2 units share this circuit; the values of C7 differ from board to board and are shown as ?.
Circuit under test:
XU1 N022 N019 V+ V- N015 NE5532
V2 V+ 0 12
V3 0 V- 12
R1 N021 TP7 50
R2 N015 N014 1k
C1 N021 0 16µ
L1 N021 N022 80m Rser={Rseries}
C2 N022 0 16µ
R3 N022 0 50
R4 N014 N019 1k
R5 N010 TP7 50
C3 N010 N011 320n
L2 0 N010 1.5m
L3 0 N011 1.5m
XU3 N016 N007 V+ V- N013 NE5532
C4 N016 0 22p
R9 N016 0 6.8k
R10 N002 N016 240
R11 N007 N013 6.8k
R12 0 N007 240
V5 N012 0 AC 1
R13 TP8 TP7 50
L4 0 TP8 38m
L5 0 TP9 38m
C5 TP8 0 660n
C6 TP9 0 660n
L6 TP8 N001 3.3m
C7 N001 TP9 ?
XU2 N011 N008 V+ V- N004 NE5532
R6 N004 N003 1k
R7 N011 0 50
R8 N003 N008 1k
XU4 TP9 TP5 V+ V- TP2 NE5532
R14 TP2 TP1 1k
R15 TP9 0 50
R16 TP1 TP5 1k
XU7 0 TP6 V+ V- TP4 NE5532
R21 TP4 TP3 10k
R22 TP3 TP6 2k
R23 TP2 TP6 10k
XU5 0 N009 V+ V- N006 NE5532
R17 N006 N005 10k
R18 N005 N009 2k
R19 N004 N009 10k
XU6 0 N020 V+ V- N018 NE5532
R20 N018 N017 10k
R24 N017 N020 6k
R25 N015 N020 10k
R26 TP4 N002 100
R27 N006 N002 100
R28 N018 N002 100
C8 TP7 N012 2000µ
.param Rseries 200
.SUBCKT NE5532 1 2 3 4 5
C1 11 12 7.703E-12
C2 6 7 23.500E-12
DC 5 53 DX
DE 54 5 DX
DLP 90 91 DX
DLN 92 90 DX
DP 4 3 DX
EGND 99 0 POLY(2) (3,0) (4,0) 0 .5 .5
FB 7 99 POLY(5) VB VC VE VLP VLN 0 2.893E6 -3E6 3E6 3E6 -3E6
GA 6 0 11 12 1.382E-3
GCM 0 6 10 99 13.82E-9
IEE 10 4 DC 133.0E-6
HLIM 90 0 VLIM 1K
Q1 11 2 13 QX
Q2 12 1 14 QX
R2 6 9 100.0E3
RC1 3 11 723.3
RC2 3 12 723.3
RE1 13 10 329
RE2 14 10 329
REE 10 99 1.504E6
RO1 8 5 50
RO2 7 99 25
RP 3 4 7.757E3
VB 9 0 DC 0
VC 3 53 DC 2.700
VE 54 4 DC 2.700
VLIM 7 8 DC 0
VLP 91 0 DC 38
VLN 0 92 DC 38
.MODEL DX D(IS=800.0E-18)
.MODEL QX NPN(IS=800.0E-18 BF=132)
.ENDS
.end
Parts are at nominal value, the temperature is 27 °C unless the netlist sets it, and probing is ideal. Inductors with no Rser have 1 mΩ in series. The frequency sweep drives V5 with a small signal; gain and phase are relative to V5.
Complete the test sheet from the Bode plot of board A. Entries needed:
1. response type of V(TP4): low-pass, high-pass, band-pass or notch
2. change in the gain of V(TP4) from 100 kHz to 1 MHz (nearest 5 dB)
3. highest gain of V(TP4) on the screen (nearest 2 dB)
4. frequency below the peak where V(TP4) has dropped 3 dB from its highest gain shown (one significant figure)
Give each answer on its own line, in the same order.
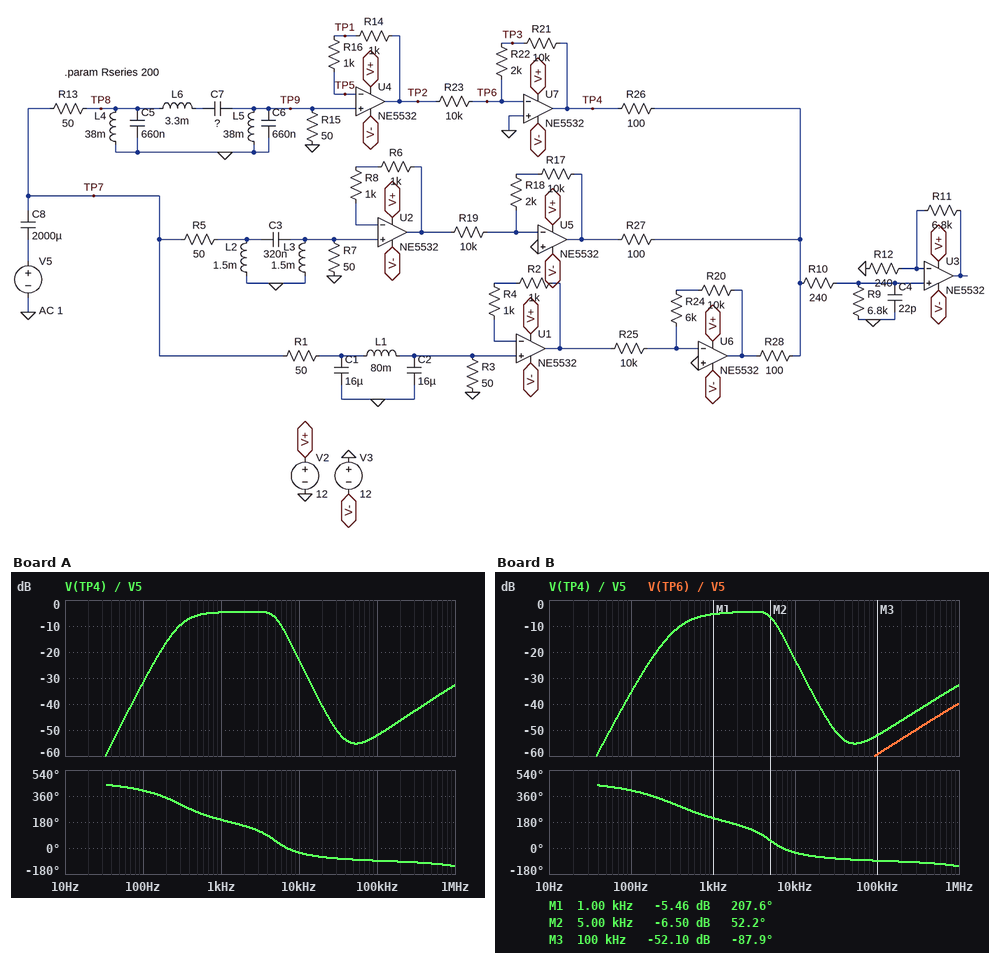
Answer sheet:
band-pass
20 dB
-4 dB
400 Hz
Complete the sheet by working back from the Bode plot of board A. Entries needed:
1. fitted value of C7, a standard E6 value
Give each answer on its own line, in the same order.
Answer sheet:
3.3 µF
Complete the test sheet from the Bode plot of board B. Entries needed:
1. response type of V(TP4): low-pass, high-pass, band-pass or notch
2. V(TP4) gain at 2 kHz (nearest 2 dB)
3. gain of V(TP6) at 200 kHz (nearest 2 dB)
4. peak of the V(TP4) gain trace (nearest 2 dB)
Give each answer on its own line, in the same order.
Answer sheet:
band-pass
-4 dB
-54 dB
-4 dB
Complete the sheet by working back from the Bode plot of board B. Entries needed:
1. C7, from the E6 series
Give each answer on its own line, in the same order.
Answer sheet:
2.2 µF
